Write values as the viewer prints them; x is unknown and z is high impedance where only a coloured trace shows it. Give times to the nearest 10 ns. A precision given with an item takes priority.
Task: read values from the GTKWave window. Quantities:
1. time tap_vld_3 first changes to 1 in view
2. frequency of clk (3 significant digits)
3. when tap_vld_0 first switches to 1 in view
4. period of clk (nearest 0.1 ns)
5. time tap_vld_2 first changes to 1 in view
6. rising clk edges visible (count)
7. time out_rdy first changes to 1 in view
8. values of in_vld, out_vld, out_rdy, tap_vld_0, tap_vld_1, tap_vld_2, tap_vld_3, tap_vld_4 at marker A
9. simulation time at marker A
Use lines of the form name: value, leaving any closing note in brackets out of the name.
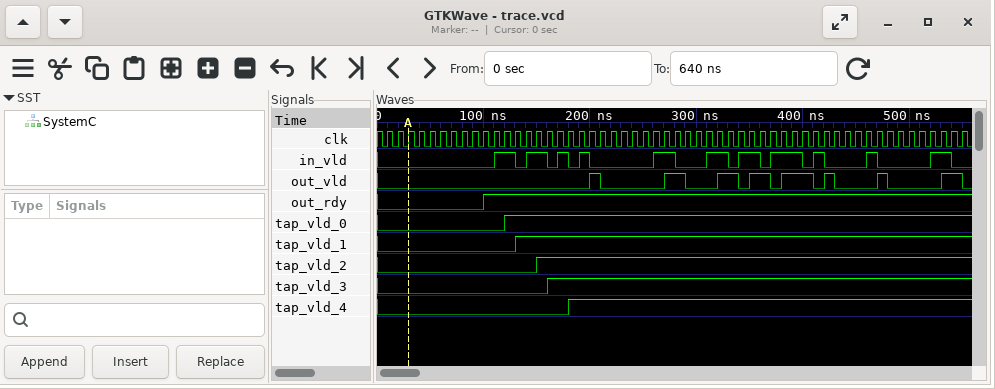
time tap_vld_3 first changes to 1 in view: 160 ns
frequency of clk: 100 MHz
when tap_vld_0 first switches to 1 in view: 120 ns
period of clk: 10 ns
time tap_vld_2 first changes to 1 in view: 150 ns
rising clk edges visible: 55
time out_rdy first changes to 1 in view: 100 ns
values of in_vld, out_vld, out_rdy, tap_vld_0, tap_vld_1, tap_vld_2, tap_vld_3, tap_vld_4 at marker A: in_vld=0, out_vld=0, out_rdy=0, tap_vld_0=0, tap_vld_1=0, tap_vld_2=0, tap_vld_3=0, tap_vld_4=0
simulation time at marker A: 30 ns
